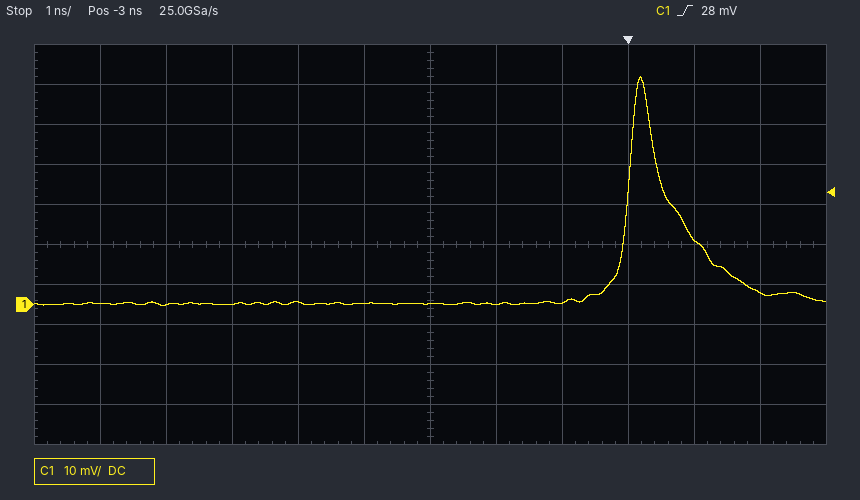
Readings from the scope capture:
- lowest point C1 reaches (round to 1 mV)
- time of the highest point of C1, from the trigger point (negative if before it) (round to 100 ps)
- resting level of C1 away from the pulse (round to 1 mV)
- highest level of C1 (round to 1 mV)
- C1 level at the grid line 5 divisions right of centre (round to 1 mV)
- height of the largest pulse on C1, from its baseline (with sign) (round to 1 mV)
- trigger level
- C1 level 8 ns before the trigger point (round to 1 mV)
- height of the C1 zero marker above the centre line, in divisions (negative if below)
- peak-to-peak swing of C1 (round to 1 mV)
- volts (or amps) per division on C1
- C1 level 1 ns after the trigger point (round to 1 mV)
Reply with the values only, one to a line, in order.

0 mV
+200 ps
0 mV
57 mV
3 mV
+57 mV
28 mV
0 mV
-1.5 div
57 mV
10 mV
16 mV
